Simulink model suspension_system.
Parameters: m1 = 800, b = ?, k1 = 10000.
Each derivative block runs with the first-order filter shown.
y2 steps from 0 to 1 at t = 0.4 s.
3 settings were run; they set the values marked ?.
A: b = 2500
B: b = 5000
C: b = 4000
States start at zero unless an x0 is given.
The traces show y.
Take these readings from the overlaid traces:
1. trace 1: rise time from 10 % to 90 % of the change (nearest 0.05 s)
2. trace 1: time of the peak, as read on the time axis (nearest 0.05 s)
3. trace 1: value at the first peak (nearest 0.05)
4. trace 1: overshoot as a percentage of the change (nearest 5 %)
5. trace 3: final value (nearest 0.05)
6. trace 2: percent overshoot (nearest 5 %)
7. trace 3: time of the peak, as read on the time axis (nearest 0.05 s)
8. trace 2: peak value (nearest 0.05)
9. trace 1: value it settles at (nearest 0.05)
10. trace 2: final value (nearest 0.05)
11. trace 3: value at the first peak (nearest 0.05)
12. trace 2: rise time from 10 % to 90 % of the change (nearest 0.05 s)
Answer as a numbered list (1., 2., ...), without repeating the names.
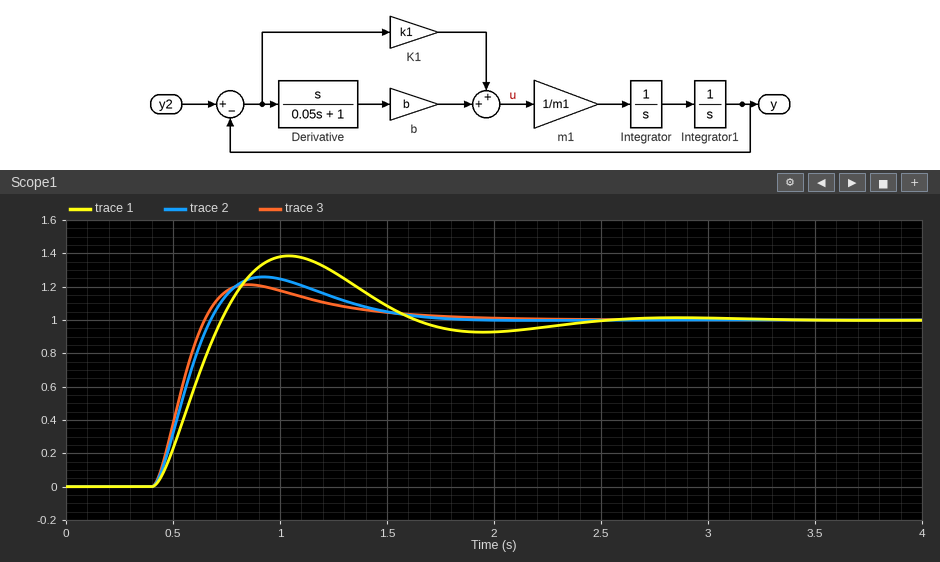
1. 0.25 s
2. 1.05 s
3. 1.40
4. 40 %
5. 1.00
6. 25 %
7. 0.85 s
8. 1.25
9. 1.00
10. 1.00
11. 1.20
12. 0.20 s
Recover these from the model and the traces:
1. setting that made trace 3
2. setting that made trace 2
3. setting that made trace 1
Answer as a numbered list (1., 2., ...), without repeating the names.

1. B
2. C
3. A
